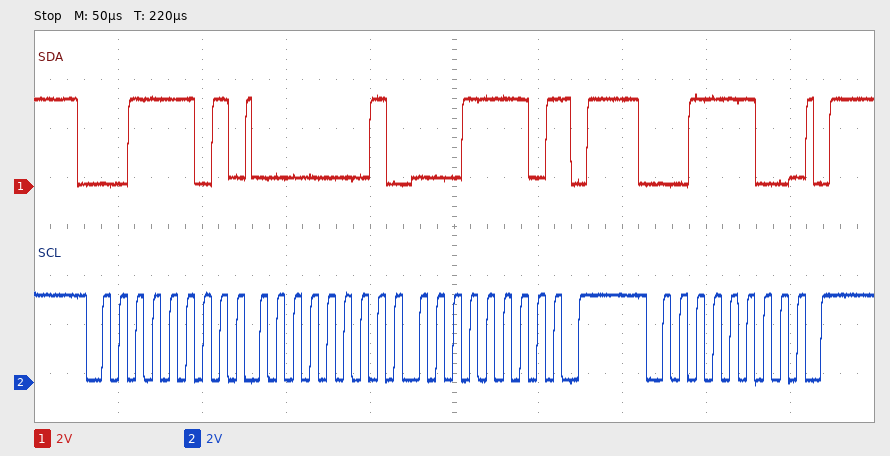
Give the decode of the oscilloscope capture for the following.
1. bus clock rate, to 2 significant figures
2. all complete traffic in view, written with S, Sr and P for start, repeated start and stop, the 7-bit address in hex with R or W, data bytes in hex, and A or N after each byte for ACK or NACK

100 kHz
S 1ER A 01 A 1E N P S 1EW A P
